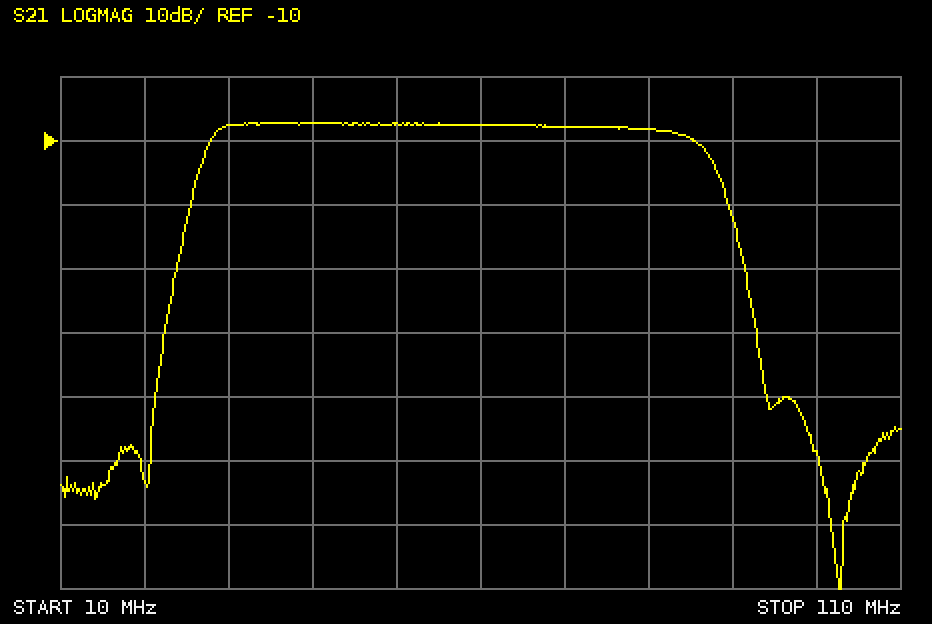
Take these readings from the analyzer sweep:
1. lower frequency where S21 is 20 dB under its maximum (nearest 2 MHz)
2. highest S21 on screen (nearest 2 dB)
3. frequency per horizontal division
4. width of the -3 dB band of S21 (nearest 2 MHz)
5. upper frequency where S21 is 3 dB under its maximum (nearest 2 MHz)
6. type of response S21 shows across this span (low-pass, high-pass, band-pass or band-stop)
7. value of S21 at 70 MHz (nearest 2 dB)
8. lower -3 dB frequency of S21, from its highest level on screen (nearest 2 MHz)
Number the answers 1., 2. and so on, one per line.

1. 24 MHz
2. -8 dB
3. 10 MHz
4. 58 MHz
5. 86 MHz
6. band-pass
7. -8 dB
8. 28 MHz
